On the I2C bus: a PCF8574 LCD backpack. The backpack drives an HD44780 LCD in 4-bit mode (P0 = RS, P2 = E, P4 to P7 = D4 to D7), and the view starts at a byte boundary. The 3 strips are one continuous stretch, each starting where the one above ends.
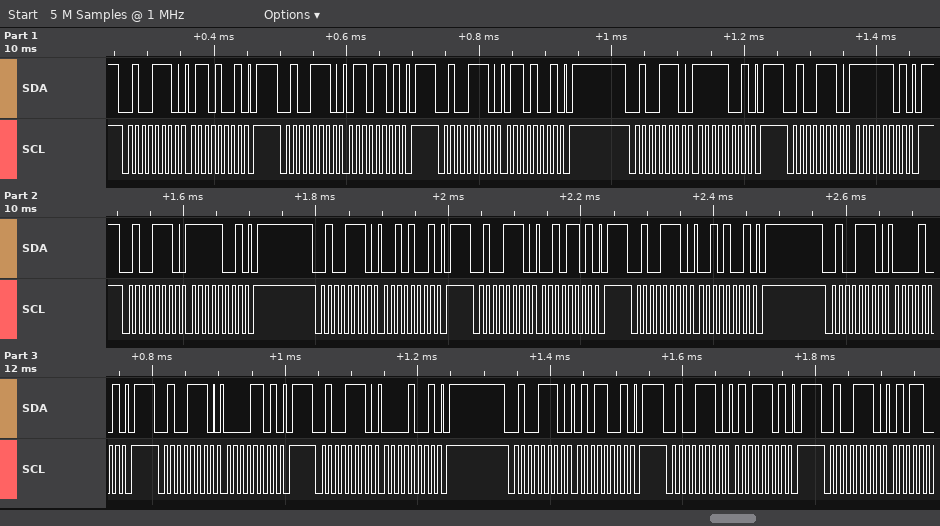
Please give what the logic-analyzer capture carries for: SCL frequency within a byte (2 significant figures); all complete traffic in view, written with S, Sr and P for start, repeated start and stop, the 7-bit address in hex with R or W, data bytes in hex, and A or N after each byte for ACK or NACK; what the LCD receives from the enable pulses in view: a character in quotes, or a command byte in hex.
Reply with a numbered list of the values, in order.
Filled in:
1. 100 kHz
2. S 27W A 69 A P S 27W A 6D A P S 27W A 69 A P S 27W A F9 A P S 27W A FD A P S 27W A F9 A P S 27W A 29 A P S 27W A 2D A P S 27W A 29 A P S 27W A 09 A P S 27W A 0D A P S 27W A 09 A P S 27W A 59 A P S 27W A 5D A P S 27W A
3. 'o' ' '
